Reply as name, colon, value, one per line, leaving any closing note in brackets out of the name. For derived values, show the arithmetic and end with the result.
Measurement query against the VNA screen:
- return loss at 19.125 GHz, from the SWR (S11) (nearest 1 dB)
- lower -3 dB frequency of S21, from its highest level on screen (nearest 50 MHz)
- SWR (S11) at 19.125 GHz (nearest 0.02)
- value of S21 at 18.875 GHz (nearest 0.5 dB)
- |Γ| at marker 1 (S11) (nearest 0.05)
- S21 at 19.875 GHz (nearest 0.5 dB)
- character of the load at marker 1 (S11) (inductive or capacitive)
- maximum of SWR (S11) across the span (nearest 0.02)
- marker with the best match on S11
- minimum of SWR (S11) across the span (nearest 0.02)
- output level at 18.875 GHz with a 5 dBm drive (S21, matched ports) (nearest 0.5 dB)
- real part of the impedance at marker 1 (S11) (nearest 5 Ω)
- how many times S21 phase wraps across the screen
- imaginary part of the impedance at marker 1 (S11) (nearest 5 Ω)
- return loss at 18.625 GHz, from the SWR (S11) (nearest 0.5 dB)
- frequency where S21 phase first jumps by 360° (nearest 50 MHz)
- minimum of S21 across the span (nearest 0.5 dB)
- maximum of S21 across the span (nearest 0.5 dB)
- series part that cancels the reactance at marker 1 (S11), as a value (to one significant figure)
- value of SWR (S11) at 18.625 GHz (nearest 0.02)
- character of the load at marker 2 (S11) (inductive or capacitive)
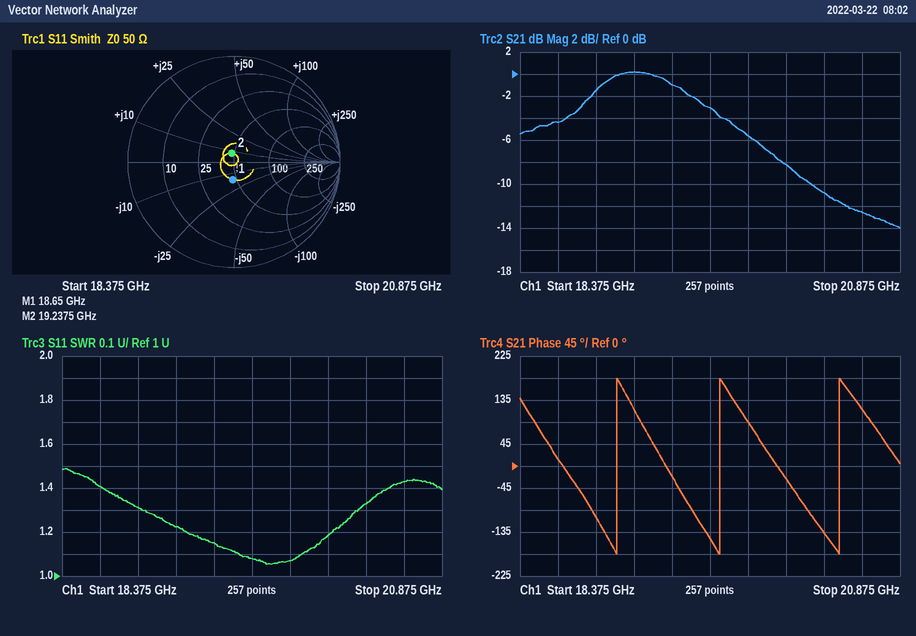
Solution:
return loss at 19.125 GHz, from the SWR (S11): −20 log10((1.22 − 1)/(1.22 + 1)) ≈ 20 dB
lower -3 dB frequency of S21, from its highest level on screen: 18.80 GHz
SWR (S11) at 19.125 GHz: 1.22
value of S21 at 18.875 GHz: -1.5 dB
|Γ| at marker 1 (S11): 0.15
S21 at 19.875 GHz: -5.5 dB
character of the load at marker 1 (S11): capacitive
maximum of SWR (S11) across the span: 1.48
marker with the best match on S11: marker 2
minimum of SWR (S11) across the span: 1.06
output level at 18.875 GHz with a 5 dBm drive (S21, matched ports): 5 dBm + (-1.5 dB) = 3.5 dBm
real part of the impedance at marker 1 (S11): 45 Ω
how many times S21 phase wraps across the screen: 3
imaginary part of the impedance at marker 1 (S11): -15 Ω
return loss at 18.625 GHz, from the SWR (S11): −20 log10((1.4 − 1)/(1.4 + 1)) ≈ 15.6 dB, so 15.5 dB to the nearest 0.5 dB
frequency where S21 phase first jumps by 360°: 19.00 GHz
minimum of S21 across the span: -14.0 dB
maximum of S21 across the span: 0.0 dB
series part that cancels the reactance at marker 1 (S11), as a value: L = 15 Ω/(2π × 18.65 GHz) ≈ 128 pH, so 100 pH to one significant figure
value of SWR (S11) at 18.625 GHz: 1.40
character of the load at marker 2 (S11): inductive
